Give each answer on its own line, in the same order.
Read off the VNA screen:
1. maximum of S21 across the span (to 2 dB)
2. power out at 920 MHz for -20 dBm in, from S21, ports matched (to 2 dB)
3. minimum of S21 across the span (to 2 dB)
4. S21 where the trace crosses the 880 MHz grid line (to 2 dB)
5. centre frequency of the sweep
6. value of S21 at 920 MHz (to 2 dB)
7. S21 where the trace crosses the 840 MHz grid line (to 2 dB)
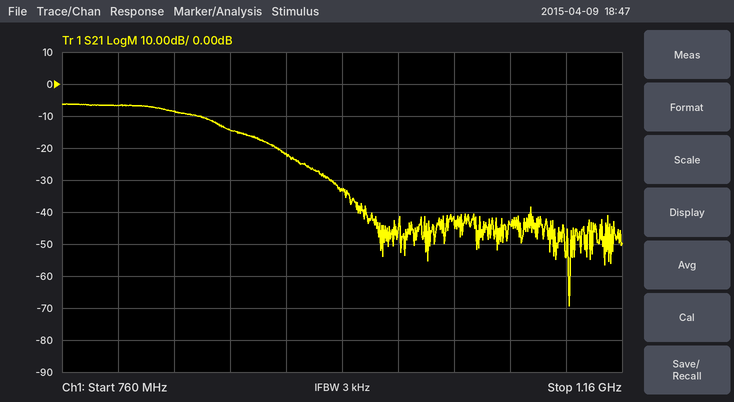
-6 dB
-42 dBm
-70 dB
-14 dB
960 MHz
-22 dB
-8 dB
